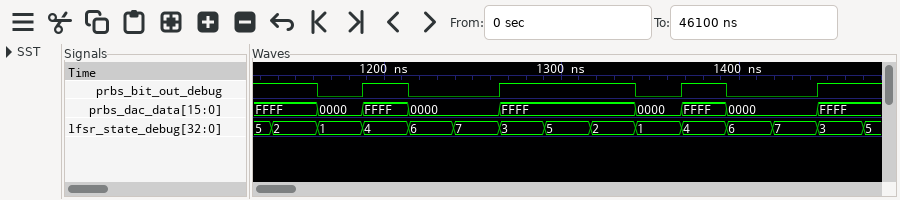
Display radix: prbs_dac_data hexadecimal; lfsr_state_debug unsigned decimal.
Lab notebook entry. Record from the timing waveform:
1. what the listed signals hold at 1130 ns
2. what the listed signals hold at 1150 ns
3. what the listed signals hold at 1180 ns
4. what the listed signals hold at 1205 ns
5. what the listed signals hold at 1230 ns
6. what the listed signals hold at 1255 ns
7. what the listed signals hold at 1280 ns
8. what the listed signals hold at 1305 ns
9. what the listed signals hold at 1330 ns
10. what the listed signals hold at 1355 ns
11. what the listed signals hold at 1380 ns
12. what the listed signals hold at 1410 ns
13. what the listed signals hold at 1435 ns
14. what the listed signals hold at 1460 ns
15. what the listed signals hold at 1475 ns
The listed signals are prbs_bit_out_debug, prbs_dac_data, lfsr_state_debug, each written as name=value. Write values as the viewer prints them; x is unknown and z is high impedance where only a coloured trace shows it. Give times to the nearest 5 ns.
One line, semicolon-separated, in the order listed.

prbs_bit_out_debug=1, prbs_dac_data=FFFF, lfsr_state_debug=5; prbs_bit_out_debug=1, prbs_dac_data=FFFF, lfsr_state_debug=2; prbs_bit_out_debug=0, prbs_dac_data=0000, lfsr_state_debug=1; prbs_bit_out_debug=1, prbs_dac_data=FFFF, lfsr_state_debug=4; prbs_bit_out_debug=0, prbs_dac_data=0000, lfsr_state_debug=6; prbs_bit_out_debug=0, prbs_dac_data=0000, lfsr_state_debug=7; prbs_bit_out_debug=1, prbs_dac_data=FFFF, lfsr_state_debug=3; prbs_bit_out_debug=1, prbs_dac_data=FFFF, lfsr_state_debug=5; prbs_bit_out_debug=1, prbs_dac_data=FFFF, lfsr_state_debug=2; prbs_bit_out_debug=0, prbs_dac_data=0000, lfsr_state_debug=1; prbs_bit_out_debug=1, prbs_dac_data=FFFF, lfsr_state_debug=4; prbs_bit_out_debug=0, prbs_dac_data=0000, lfsr_state_debug=6; prbs_bit_out_debug=0, prbs_dac_data=0000, lfsr_state_debug=7; prbs_bit_out_debug=1, prbs_dac_data=FFFF, lfsr_state_debug=3; prbs_bit_out_debug=1, prbs_dac_data=FFFF, lfsr_state_debug=5
